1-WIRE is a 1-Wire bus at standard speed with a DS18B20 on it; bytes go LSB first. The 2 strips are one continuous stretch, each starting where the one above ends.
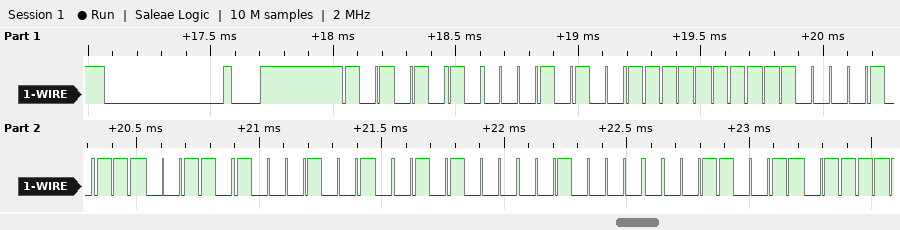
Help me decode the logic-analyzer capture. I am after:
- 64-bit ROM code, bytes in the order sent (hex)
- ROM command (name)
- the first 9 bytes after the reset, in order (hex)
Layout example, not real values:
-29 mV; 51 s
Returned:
28 FF 43 67 91 14 04 CC; Match ROM; 55 28 FF 43 67 91 14 04 CC
